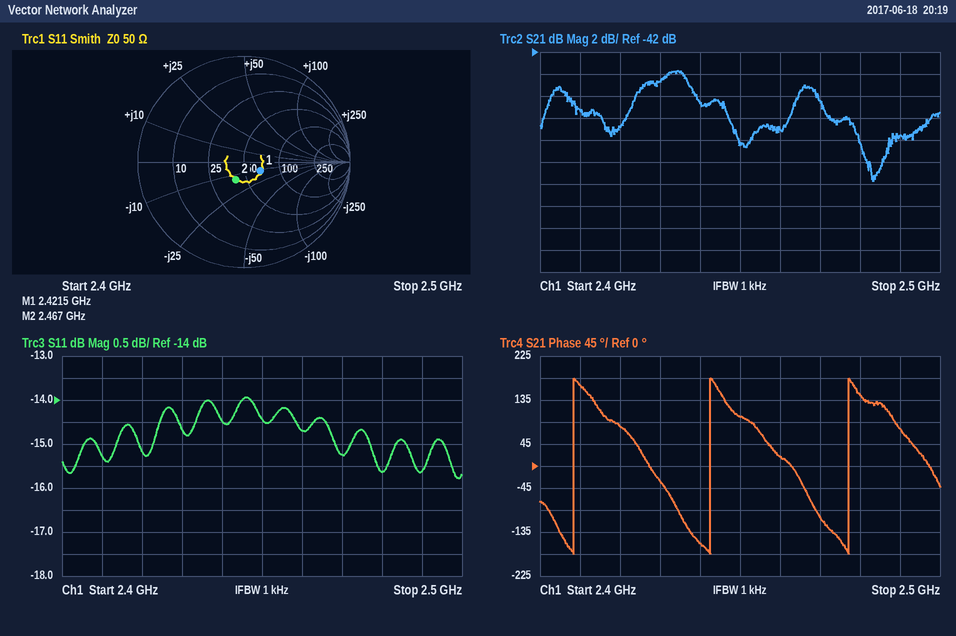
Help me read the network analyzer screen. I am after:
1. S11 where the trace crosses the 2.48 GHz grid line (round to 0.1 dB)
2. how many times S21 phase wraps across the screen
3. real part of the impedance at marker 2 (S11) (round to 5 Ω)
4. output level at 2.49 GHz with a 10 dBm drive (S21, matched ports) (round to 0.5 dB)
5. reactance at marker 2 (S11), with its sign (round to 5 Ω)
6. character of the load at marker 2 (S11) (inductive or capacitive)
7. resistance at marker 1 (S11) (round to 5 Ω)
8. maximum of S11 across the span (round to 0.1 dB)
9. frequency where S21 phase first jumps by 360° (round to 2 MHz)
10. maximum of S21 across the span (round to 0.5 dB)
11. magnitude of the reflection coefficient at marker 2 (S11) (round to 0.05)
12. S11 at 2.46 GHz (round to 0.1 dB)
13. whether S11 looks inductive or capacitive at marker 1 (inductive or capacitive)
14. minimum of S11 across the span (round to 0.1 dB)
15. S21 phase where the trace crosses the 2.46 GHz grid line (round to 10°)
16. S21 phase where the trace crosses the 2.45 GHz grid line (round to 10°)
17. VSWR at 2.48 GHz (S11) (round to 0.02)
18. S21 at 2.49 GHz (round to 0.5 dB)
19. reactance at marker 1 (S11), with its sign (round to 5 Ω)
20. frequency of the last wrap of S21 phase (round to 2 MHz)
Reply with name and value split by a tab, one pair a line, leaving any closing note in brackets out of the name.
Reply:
S11 where the trace crosses the 2.48 GHz grid line	-15.6 dB
how many times S21 phase wraps across the screen	3
real part of the impedance at marker 2 (S11)	40 Ω
output level at 2.49 GHz with a 10 dBm drive (S21, matched ports)	-39.5 dBm
reactance at marker 2 (S11), with its sign	-15 Ω
character of the load at marker 2 (S11)	capacitive
resistance at marker 1 (S11)	65 Ω
maximum of S11 across the span	-13.9 dB
frequency where S21 phase first jumps by 360°	2.408 GHz
maximum of S21 across the span	-43.5 dB
magnitude of the reflection coefficient at marker 2 (S11)	0.20
S11 at 2.46 GHz	-14.7 dB
whether S11 looks inductive or capacitive at marker 1	capacitive
minimum of S11 across the span	-15.8 dB
S21 phase where the trace crosses the 2.46 GHz grid line	20°
S21 phase where the trace crosses the 2.45 GHz grid line	100°
VSWR at 2.48 GHz (S11)	1.40
S21 at 2.49 GHz	-49.5 dB
reactance at marker 1 (S11), with its sign	-10 Ω
frequency of the last wrap of S21 phase	2.478 GHz
